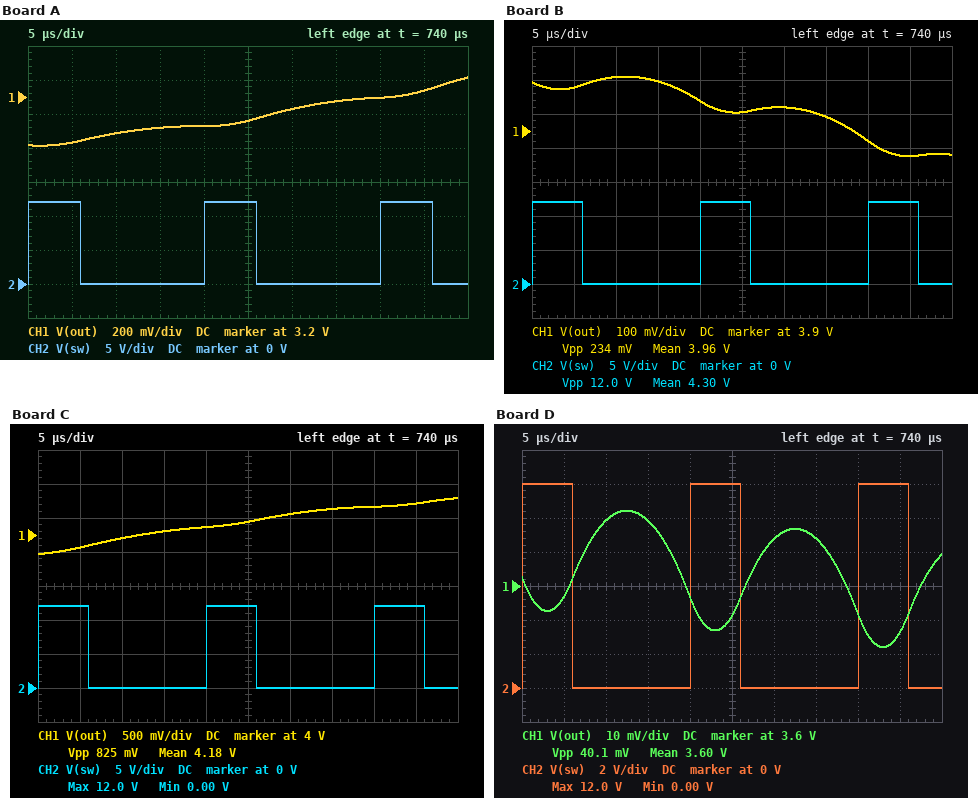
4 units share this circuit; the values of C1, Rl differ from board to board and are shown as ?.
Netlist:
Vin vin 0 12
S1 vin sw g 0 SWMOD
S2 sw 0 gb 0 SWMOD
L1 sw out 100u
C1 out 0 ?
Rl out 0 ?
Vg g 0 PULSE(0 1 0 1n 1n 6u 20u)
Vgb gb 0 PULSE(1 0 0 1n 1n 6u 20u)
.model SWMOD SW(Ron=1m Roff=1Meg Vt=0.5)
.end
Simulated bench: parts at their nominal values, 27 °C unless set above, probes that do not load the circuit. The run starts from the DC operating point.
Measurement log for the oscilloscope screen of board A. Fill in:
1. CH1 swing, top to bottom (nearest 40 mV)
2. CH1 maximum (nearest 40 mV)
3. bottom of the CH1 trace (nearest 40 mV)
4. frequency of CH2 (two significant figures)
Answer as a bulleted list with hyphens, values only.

- 400 mV
- 3.32 V
- 2.92 V
- 50 kHz
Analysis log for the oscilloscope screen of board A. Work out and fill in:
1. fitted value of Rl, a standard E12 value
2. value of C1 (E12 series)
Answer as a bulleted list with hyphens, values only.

- 6.8 Ω
- 33 µF
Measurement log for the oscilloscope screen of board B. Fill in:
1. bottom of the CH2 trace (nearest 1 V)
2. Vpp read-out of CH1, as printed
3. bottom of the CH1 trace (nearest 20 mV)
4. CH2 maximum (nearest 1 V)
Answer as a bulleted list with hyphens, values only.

- 0 V
- 234 mV
- 3.82 V
- 12 V
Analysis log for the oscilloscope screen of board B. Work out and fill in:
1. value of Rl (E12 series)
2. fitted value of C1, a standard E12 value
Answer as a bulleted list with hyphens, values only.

- 8.2 Ω
- 22 µF
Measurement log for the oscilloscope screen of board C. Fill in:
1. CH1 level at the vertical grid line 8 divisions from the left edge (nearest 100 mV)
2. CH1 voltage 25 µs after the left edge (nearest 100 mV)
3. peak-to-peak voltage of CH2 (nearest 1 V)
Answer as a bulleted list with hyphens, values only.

- 4.4 V
- 4.2 V
- 12 V
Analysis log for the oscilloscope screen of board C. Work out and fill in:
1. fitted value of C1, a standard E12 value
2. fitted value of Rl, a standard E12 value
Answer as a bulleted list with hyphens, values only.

- 27 µF
- 12 Ω
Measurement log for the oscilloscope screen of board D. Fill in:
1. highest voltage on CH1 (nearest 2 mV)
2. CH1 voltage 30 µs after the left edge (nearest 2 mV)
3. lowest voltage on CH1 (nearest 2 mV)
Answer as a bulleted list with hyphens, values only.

- 3.622 V
- 3.614 V
- 3.582 V
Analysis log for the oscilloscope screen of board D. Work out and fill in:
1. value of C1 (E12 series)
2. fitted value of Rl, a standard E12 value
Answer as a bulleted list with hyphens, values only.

- 39 µF
- 1.8 Ω
